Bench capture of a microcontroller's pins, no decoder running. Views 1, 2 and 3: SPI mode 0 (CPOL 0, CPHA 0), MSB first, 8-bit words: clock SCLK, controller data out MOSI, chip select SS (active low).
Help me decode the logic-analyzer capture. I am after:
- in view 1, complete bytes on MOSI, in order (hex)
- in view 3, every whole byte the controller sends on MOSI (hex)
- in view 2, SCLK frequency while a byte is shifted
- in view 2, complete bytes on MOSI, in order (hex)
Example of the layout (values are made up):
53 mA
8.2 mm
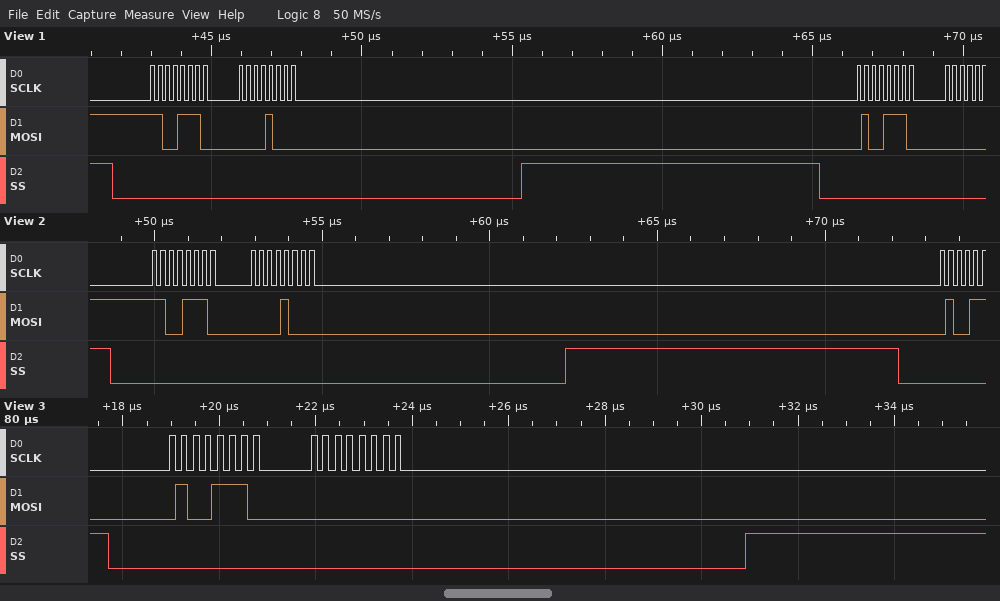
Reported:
CE 08 4E
4E 00
4 MHz
0xCE 0x08
